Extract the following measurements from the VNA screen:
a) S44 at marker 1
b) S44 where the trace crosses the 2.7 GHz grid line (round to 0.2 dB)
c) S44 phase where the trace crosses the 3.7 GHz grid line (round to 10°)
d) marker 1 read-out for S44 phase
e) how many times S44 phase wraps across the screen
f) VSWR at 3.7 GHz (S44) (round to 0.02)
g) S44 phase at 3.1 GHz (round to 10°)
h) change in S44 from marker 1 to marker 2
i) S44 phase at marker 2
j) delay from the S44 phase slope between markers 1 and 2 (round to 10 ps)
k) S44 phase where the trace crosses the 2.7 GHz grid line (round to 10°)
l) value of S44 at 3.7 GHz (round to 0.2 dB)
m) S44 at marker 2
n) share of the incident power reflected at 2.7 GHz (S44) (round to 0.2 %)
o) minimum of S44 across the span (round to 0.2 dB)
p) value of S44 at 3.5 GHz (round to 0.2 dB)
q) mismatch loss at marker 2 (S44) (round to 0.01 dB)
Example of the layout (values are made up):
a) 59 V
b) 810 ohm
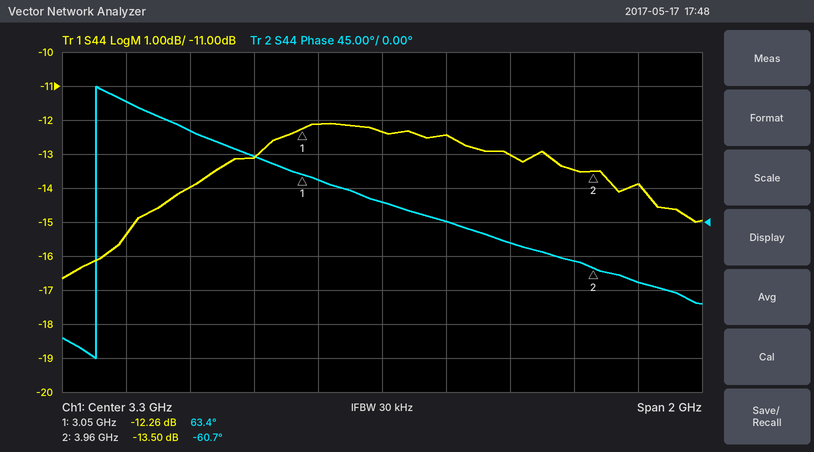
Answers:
a) -12.26 dB
b) -14.0 dB
c) -30°
d) 63.4°
e) 1
f) 1.58
g) 60°
h) -1.24 dB
i) -60.7°
j) 380 ps
k) 120°
l) -13.0 dB
m) -13.50 dB
n) 4.0 %
o) -16.6 dB
p) -12.4 dB
q) 0.20 dB
